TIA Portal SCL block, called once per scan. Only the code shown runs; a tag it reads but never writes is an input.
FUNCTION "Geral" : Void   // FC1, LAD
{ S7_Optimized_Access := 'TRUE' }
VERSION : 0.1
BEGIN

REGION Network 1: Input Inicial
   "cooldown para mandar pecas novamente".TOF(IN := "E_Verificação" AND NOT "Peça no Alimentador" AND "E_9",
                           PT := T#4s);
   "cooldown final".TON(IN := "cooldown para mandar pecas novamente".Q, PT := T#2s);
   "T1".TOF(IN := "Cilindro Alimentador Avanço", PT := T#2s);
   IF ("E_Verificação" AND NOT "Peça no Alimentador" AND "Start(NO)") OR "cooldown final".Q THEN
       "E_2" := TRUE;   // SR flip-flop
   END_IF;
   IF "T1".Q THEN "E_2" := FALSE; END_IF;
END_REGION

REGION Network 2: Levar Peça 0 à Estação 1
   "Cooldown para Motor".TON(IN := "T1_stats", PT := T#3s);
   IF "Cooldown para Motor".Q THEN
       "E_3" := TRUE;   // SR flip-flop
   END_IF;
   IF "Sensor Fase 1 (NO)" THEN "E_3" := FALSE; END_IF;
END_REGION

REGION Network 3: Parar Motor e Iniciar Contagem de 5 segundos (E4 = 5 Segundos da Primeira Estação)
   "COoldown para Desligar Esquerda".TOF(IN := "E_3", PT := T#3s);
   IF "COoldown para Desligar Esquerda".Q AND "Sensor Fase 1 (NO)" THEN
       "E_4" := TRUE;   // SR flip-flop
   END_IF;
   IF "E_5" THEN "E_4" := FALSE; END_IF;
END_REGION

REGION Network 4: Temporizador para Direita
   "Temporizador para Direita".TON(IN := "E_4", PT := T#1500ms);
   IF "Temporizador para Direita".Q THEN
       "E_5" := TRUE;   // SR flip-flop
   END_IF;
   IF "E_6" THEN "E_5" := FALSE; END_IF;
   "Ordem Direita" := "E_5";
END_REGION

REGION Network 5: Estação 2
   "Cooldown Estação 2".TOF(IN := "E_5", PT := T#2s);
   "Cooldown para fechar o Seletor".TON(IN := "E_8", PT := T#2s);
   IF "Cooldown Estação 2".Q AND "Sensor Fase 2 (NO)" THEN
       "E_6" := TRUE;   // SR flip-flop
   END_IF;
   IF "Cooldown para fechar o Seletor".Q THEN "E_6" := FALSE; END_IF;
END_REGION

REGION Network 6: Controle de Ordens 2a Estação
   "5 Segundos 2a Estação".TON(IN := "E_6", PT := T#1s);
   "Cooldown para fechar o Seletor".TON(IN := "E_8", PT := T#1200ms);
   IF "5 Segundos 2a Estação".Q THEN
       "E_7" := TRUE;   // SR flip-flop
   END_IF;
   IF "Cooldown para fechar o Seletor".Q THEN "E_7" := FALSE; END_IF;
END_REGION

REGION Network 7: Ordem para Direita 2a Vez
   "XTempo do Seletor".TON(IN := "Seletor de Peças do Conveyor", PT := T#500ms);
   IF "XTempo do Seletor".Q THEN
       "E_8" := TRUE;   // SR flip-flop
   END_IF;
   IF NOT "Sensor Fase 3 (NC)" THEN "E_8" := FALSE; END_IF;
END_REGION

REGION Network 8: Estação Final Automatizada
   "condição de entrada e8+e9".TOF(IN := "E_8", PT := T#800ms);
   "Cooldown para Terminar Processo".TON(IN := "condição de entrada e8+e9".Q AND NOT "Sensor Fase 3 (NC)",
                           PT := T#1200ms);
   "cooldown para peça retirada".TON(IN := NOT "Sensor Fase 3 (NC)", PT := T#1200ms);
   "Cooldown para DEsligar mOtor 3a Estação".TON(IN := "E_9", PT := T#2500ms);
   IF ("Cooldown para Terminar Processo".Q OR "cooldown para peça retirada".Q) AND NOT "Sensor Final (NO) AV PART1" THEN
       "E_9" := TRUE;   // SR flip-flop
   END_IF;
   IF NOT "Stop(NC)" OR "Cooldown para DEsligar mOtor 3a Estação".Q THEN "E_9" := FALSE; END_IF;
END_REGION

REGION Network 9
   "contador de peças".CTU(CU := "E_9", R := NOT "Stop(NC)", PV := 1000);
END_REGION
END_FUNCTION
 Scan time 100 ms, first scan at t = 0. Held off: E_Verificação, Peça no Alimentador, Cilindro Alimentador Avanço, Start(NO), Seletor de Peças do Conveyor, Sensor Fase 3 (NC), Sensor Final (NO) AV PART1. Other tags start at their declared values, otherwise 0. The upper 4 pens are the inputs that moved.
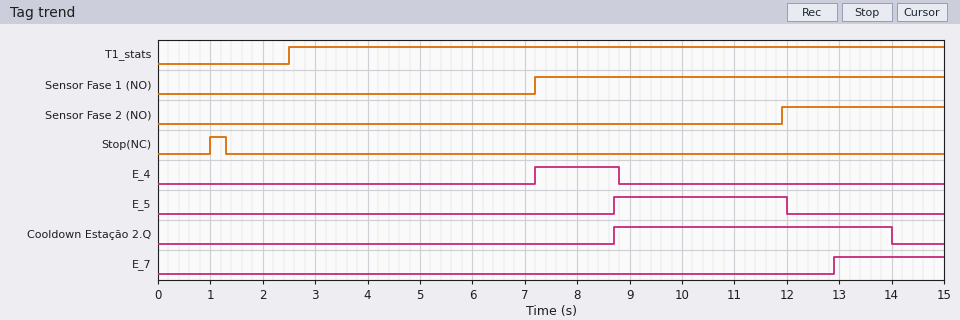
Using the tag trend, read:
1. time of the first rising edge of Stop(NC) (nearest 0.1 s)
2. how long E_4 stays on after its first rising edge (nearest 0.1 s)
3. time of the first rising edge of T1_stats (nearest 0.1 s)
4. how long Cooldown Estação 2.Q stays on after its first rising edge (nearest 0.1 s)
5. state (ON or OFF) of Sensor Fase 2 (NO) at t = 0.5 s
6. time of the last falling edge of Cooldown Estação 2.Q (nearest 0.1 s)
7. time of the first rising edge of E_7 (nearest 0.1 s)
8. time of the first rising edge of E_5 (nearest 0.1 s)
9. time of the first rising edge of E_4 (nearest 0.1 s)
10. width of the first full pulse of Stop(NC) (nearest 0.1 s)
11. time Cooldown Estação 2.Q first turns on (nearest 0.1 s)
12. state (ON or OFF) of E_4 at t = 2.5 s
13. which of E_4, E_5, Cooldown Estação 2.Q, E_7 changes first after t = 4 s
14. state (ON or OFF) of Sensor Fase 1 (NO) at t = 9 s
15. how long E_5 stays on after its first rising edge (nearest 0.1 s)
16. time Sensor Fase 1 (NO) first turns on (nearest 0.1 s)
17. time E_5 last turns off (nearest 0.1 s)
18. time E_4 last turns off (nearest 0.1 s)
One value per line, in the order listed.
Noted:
1.0 s
1.6 s
2.5 s
5.3 s
OFF
14.0 s
12.9 s
8.7 s
7.2 s
0.3 s
8.7 s
OFF
E_4
ON
3.3 s
7.2 s
12.0 s
8.8 s
